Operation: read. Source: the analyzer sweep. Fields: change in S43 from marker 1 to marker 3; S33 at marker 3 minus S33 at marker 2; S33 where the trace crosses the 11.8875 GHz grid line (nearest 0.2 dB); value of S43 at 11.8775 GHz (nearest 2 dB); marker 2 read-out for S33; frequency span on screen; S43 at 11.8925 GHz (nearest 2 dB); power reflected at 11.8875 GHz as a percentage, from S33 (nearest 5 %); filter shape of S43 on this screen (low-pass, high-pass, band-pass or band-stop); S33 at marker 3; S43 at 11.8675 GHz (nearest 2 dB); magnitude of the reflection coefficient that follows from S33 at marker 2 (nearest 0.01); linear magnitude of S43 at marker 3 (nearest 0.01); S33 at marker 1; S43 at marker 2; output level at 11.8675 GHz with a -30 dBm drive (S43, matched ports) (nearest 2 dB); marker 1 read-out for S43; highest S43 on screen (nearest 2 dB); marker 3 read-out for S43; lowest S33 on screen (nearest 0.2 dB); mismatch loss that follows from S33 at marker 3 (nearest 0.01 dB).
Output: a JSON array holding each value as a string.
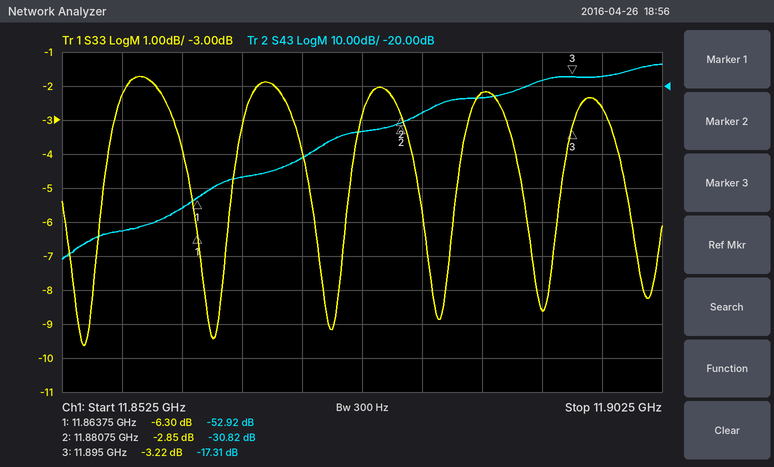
["35.61 dB", "-0.37 dB", "-2.2 dB", "-34 dB", "-2.85 dB", "50 MHz", "-18 dB", "60 %", "high-pass", "-3.22 dB", "-46 dB", "0.72", "0.14", "-6.30 dB", "-30.82 dB", "-76 dBm", "-52.92 dB", "-14 dB", "-17.31 dB", "-9.6 dB", "2.81 dB"]
